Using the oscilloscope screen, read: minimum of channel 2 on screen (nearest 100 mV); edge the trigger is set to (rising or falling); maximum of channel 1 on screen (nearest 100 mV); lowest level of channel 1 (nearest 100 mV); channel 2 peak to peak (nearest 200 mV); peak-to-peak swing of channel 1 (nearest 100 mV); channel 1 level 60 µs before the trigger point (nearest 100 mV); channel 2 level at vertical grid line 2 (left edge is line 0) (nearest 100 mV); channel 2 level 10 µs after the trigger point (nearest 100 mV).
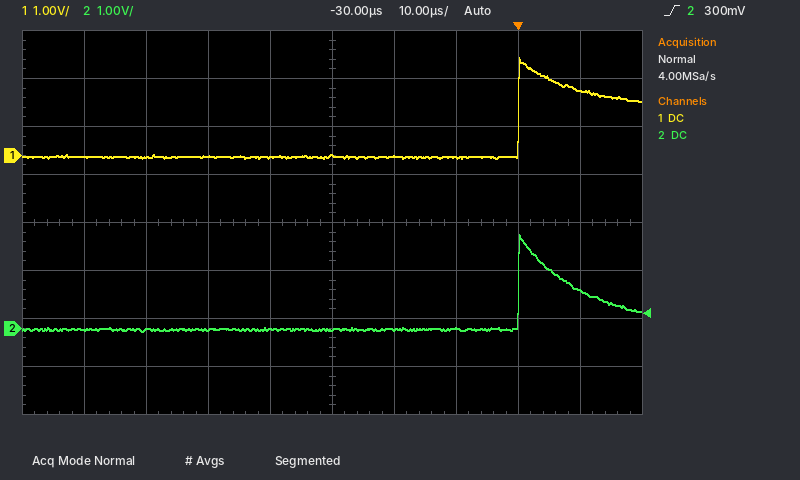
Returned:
-100 mV
rising
2.0 V
-100 mV
2.0 V
2.1 V
0.0 V
0.0 V
800 mV
